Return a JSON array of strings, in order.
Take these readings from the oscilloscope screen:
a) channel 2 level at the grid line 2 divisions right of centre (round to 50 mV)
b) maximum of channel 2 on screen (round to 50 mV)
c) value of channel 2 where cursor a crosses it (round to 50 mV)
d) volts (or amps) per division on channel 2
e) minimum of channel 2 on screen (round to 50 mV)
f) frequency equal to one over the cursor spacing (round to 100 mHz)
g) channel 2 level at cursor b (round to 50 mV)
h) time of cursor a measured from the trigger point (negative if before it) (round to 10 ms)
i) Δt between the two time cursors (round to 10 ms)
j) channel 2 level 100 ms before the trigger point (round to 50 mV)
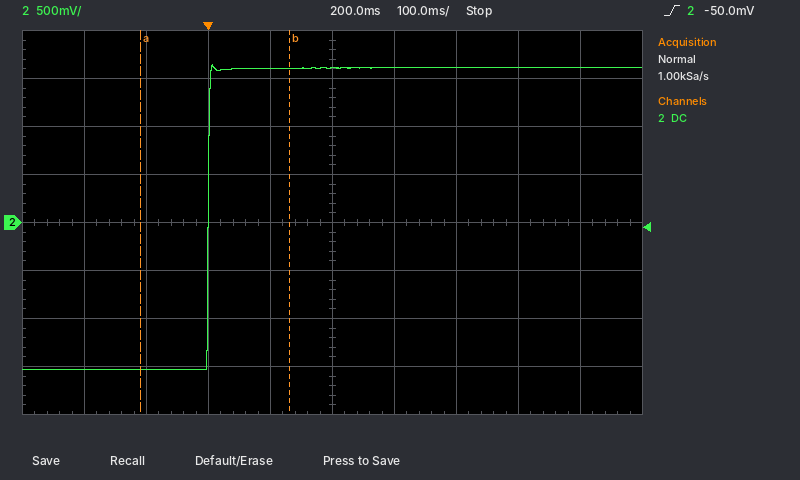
["1.60 V", "1.65 V", "-1.55 V", "500 mV", "-1.55 V", "4.2 Hz", "1.60 V", "-110 ms", "240 ms", "-1.55 V"]
